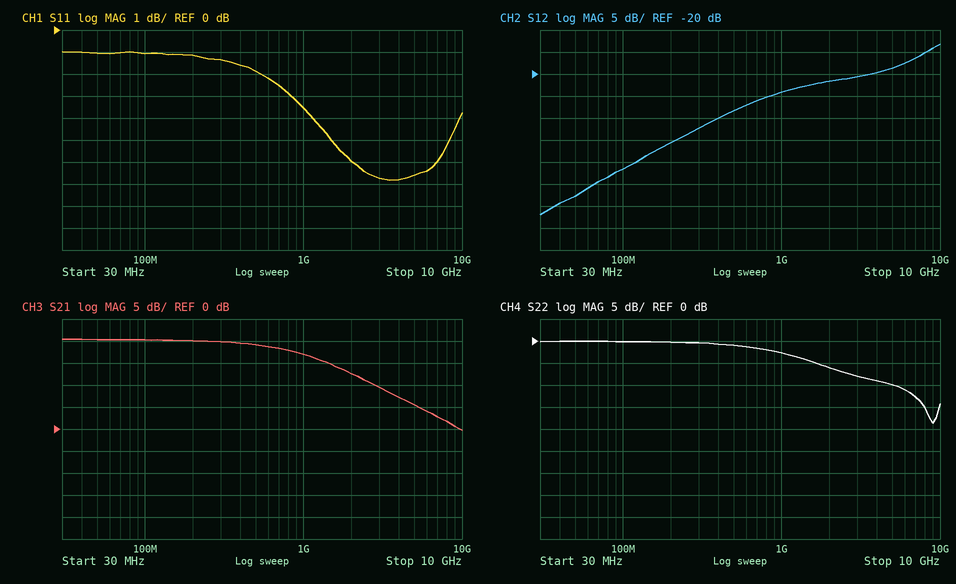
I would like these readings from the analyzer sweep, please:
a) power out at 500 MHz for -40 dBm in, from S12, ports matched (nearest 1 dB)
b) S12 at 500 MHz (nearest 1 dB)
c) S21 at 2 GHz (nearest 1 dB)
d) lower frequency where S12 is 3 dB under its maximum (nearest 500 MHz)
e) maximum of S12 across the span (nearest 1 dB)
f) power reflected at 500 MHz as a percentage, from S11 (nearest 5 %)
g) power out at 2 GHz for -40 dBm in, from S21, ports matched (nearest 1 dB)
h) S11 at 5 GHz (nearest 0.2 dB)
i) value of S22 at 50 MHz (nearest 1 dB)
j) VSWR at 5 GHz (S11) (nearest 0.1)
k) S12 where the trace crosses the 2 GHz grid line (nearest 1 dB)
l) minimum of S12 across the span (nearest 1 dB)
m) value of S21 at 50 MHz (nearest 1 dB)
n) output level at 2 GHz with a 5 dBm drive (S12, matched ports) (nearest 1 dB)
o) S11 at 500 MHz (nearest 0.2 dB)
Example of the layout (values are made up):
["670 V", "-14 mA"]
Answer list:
["-68 dBm", "-28 dB", "13 dB", "7.0 GHz", "-13 dB", "65 %", "-27 dBm", "-6.6 dB", "0 dB", "2.8", "-22 dB", "-52 dB", "20 dB", "-17 dBm", "-1.8 dB"]
